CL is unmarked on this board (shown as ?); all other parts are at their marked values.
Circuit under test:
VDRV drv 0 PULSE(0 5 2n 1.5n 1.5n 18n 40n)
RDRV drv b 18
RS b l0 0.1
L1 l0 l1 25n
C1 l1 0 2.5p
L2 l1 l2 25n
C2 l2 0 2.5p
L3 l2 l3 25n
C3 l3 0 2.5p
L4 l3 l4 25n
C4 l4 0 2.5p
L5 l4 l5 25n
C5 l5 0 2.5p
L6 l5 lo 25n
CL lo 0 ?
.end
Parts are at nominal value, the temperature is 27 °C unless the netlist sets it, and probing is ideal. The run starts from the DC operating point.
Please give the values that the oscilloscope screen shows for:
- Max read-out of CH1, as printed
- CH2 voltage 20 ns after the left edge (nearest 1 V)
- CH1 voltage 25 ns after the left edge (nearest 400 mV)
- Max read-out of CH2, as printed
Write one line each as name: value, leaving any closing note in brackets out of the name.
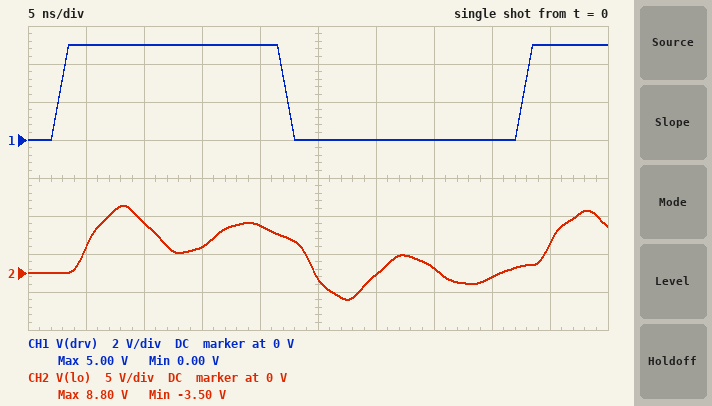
Max read-out of CH1, as printed: 5.00 V
CH2 voltage 20 ns after the left edge: 6 V
CH1 voltage 25 ns after the left edge: 0 V
Max read-out of CH2, as printed: 8.80 V
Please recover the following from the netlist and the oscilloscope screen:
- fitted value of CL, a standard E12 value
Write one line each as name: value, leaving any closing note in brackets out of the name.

fitted value of CL, a standard E12 value: 15 pF
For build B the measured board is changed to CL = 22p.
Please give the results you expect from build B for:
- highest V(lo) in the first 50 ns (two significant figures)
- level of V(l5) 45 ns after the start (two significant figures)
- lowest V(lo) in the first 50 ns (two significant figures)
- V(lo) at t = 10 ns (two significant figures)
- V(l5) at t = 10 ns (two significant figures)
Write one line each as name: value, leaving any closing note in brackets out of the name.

highest V(lo) in the first 50 ns: 9.3 V
level of V(l5) 45 ns after the start: 3.2 V
lowest V(lo) in the first 50 ns: -4.3 V
V(lo) at t = 10 ns: 7.8 V
V(l5) at t = 10 ns: 7.7 V
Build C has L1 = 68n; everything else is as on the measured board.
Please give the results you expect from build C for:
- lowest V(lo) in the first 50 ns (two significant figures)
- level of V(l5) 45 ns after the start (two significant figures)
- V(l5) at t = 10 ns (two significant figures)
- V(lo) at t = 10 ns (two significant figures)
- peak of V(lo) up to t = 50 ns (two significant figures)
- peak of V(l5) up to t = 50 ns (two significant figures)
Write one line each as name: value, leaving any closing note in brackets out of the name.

lowest V(lo) in the first 50 ns: -5.1 V
level of V(l5) 45 ns after the start: 3.3 V
V(l5) at t = 10 ns: 8.0 V
V(lo) at t = 10 ns: 8.4 V
peak of V(lo) up to t = 50 ns: 10 V
peak of V(l5) up to t = 50 ns: 9.5 V
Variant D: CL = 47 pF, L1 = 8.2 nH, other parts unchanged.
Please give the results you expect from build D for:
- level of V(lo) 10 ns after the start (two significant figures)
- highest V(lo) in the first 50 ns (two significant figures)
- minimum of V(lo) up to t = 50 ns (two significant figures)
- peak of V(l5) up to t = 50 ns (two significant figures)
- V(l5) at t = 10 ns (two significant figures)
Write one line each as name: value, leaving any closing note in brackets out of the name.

level of V(lo) 10 ns after the start: 7.5 V
highest V(lo) in the first 50 ns: 7.8 V
minimum of V(lo) up to t = 50 ns: -2.5 V
peak of V(l5) up to t = 50 ns: 7.6 V
V(l5) at t = 10 ns: 7.1 V
